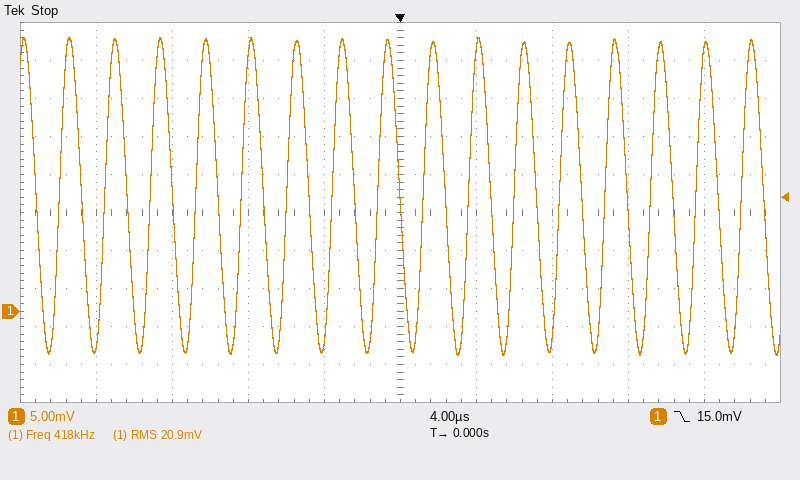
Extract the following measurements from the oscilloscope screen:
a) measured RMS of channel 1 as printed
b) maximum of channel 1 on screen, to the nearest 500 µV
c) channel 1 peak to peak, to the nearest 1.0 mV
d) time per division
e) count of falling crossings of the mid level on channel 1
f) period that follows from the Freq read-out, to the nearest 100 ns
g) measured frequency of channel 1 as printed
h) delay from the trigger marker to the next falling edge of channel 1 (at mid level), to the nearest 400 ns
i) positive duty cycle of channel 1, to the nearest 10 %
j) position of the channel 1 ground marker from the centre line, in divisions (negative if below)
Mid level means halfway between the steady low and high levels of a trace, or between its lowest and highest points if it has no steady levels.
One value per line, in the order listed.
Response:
20.9 mV
36.0 mV
42.0 mV
4 µs
17
2.4 µs
418 kHz
2.4 µs
50 %
-2.6 div
